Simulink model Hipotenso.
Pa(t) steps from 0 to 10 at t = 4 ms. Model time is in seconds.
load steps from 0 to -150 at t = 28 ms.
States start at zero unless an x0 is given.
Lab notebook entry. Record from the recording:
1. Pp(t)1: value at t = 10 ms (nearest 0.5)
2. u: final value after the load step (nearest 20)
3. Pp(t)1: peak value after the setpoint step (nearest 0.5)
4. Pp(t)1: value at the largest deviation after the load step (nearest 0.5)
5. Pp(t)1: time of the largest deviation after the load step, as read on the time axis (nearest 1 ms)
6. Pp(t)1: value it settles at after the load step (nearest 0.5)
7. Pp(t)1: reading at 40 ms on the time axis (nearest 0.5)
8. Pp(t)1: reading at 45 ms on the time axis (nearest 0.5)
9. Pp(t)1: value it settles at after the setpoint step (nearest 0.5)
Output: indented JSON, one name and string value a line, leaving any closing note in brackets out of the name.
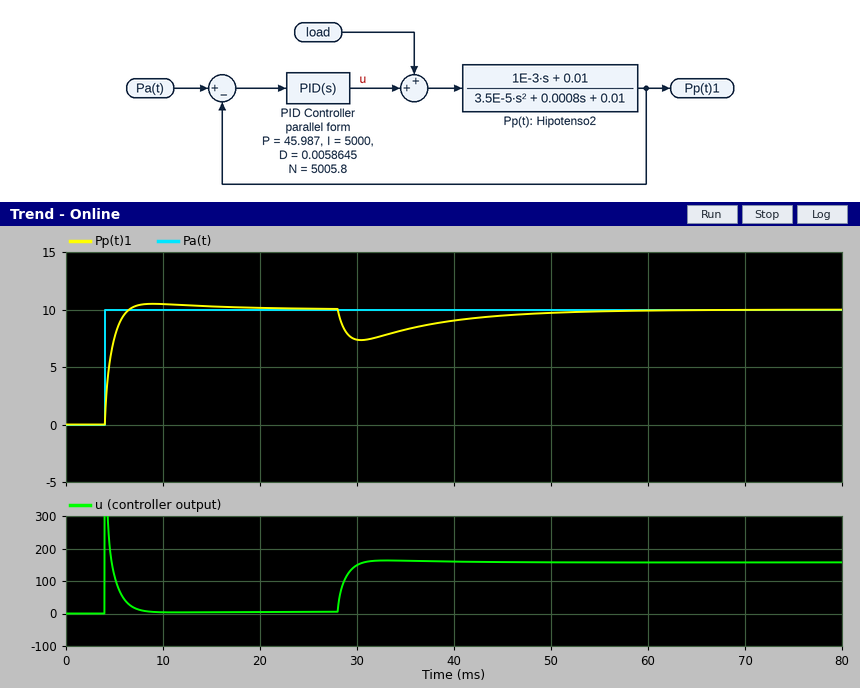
{
  "Pp(t)1: value at t = 10 ms": "10.5",
  "u: final value after the load step": "160",
  "Pp(t)1: peak value after the setpoint step": "10.5",
  "Pp(t)1: value at the largest deviation after the load step": "7.5",
  "Pp(t)1: time of the largest deviation after the load step, as read on the time axis": "30 ms",
  "Pp(t)1: value it settles at after the load step": "10.0",
  "Pp(t)1: reading at 40 ms on the time axis": "9.0",
  "Pp(t)1: reading at 45 ms on the time axis": "9.5",
  "Pp(t)1: value it settles at after the setpoint step": "10.0"
}
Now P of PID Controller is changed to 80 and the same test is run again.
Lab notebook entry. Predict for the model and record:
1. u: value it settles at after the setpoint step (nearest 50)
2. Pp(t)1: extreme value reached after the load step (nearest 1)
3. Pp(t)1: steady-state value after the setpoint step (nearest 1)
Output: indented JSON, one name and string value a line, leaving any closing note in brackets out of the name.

{
  "u: value it settles at after the setpoint step": "0",
  "Pp(t)1: extreme value reached after the load step": "8",
  "Pp(t)1: steady-state value after the setpoint step": "10"
}
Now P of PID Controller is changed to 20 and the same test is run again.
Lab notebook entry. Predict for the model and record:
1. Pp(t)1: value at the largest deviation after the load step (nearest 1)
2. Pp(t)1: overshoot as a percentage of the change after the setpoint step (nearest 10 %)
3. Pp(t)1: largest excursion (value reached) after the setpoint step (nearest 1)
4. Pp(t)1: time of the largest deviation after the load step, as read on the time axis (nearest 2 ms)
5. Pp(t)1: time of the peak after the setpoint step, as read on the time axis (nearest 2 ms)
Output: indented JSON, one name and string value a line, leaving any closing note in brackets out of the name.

{
  "Pp(t)1: value at the largest deviation after the load step": "5",
  "Pp(t)1: overshoot as a percentage of the change after the setpoint step": "20 %",
  "Pp(t)1: largest excursion (value reached) after the setpoint step": "12",
  "Pp(t)1: time of the largest deviation after the load step, as read on the time axis": "32 ms",
  "Pp(t)1: time of the peak after the setpoint step, as read on the time axis": "10 ms"
}
